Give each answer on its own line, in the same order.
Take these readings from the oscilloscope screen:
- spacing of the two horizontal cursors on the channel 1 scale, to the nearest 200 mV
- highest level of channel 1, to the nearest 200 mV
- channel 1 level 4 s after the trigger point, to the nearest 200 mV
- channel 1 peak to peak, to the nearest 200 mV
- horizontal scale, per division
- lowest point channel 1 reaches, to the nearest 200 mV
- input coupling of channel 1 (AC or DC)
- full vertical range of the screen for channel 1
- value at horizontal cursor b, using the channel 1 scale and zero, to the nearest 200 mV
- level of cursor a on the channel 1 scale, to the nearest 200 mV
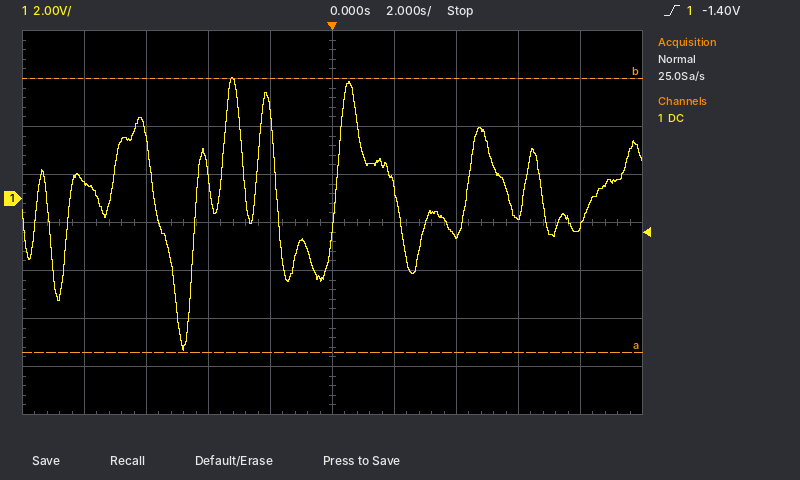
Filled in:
11.4 V
5.0 V
-1.6 V
11.4 V
2 s
-6.4 V
DC
16 V
5.0 V
-6.4 V
